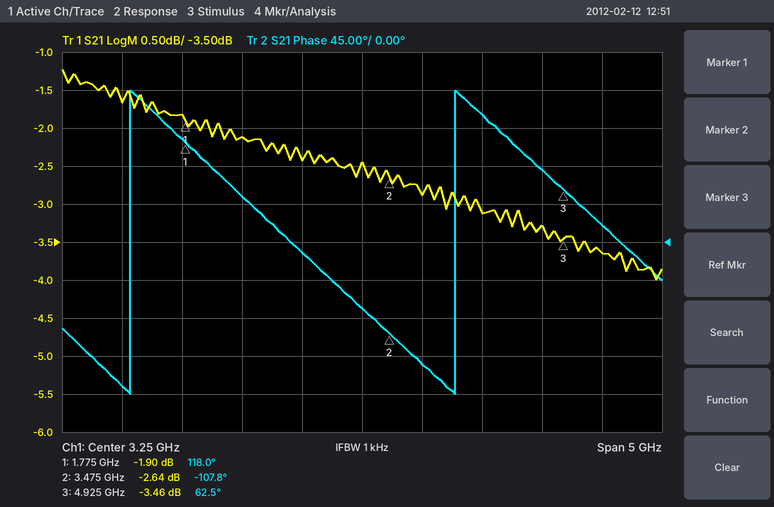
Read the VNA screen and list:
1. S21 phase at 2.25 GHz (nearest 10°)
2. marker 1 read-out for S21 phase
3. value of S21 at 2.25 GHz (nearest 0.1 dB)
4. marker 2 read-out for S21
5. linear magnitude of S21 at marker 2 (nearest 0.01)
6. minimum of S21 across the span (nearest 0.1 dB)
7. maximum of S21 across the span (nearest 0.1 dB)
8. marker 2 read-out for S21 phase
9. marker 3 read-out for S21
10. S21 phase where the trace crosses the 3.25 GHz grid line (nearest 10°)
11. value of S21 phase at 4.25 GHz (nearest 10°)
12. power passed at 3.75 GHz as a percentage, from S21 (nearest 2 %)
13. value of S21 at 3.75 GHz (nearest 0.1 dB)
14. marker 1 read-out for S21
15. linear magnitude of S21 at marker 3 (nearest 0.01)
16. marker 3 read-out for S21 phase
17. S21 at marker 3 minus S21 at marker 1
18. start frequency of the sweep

50°
118.0°
-2.1 dB
-2.64 dB
0.74
-4.0 dB
-1.2 dB
-107.8°
-3.46 dB
-80°
150°
52 %
-2.9 dB
-1.90 dB
0.67
62.5°
-1.56 dB
750 MHz
